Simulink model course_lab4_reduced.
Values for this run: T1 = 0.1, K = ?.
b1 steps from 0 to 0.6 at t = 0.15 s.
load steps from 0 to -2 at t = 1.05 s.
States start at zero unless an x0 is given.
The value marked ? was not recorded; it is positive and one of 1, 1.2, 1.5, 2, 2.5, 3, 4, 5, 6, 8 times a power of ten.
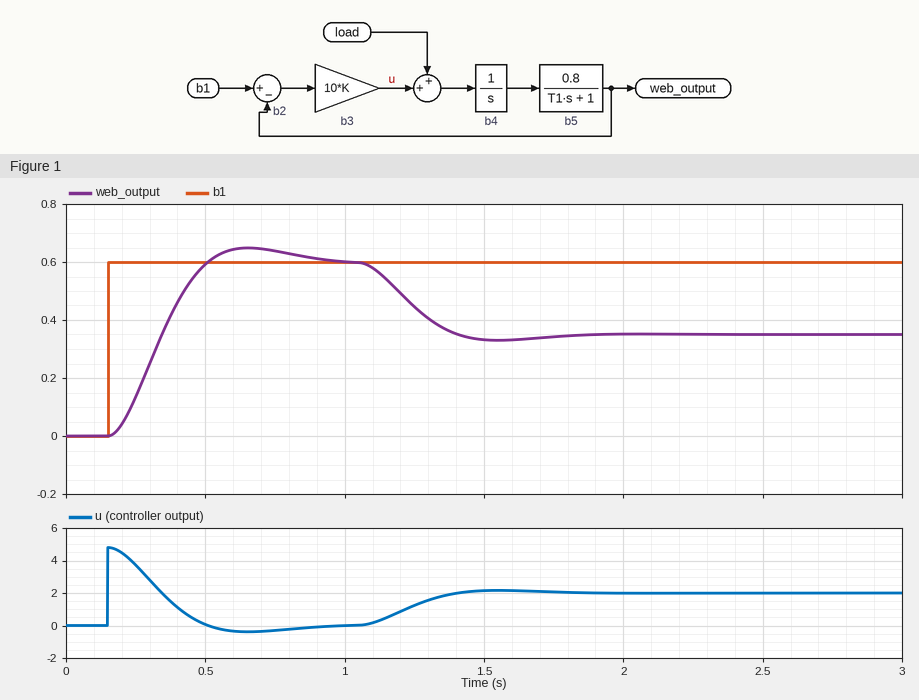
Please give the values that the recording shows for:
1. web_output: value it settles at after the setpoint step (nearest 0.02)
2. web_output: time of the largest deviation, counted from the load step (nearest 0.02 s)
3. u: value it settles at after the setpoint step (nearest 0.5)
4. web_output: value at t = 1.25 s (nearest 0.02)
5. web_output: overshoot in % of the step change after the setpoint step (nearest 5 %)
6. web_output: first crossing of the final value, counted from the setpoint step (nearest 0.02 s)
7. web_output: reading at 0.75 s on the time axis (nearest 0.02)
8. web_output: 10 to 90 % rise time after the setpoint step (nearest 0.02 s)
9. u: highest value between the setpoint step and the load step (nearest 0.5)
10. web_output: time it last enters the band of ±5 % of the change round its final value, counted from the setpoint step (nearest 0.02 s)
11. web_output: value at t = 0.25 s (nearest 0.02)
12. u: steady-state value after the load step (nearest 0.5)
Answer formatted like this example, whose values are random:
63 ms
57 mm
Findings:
0.60
0.50 s
0.0
0.44
10 %
0.36 s
0.64
0.24 s
5.0
0.64 s
0.14
2.0
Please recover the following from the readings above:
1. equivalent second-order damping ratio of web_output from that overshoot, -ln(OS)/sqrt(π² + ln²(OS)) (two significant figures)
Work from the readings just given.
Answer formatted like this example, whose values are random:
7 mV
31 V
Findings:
0.59
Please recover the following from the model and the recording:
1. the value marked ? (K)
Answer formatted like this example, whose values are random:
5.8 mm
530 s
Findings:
0.8
